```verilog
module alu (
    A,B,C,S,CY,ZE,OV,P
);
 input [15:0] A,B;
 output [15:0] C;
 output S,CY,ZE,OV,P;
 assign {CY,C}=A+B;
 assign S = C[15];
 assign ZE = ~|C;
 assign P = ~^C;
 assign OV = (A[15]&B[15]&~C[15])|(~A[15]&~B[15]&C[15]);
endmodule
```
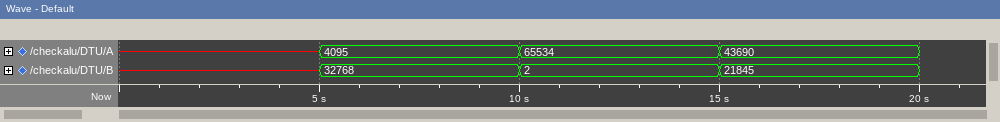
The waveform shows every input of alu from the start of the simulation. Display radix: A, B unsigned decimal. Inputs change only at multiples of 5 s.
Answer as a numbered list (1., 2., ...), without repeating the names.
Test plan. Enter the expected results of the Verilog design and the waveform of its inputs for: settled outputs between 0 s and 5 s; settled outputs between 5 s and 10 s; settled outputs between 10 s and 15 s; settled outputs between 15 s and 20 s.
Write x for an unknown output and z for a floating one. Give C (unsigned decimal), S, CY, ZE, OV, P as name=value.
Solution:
1. C=x, S=x, CY=x, ZE=x, OV=x, P=x
2. C=36863, S=1, CY=0, ZE=0, OV=0, P=0
3. C=0, S=0, CY=1, ZE=1, OV=0, P=1
4. C=65535, S=1, CY=0, ZE=0, OV=0, P=1
